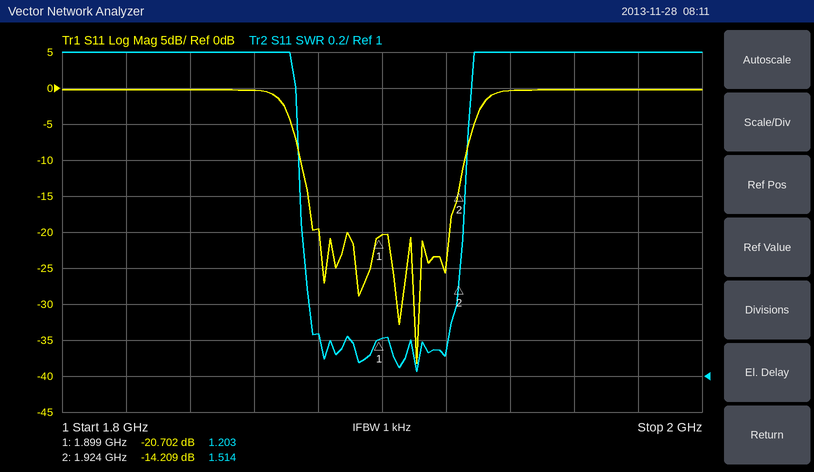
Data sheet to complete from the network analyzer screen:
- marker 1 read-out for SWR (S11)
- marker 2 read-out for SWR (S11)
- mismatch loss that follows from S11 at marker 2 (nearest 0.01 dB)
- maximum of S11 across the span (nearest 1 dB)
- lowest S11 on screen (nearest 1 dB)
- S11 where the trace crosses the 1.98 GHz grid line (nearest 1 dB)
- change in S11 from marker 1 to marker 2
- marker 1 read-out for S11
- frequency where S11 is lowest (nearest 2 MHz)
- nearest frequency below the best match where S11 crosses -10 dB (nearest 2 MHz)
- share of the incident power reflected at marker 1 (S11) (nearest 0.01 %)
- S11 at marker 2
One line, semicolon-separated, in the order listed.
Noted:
1.203; 1.514; 0.17 dB; 0 dB; -38 dB; 0 dB; 6.493 dB; -20.702 dB; 1.910 GHz; 1.874 GHz; 0.85 %; -14.209 dB
